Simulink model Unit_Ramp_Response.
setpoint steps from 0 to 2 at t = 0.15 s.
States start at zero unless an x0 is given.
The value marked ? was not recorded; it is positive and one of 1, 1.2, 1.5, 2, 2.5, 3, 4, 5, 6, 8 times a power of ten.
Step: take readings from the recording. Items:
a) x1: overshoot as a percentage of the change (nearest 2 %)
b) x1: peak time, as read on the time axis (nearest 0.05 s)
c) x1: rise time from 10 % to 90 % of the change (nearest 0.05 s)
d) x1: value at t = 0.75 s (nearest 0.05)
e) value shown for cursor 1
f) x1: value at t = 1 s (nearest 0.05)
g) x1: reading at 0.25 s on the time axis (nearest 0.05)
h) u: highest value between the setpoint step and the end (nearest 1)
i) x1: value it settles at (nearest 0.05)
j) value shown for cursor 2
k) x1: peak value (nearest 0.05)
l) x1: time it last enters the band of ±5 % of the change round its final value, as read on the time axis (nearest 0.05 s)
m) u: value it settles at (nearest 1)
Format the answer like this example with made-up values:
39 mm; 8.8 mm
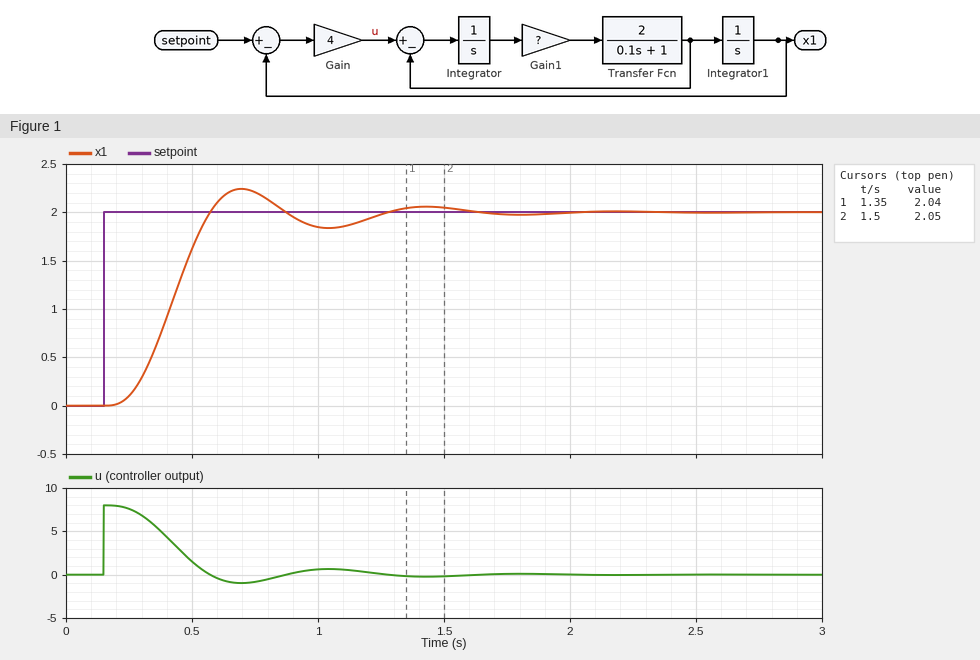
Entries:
12 %; 0.70 s; 0.25 s; 2.20; 2.04; 1.85; 0.10; 8; 2.00; 2.05; 2.25; 1.15 s; 0
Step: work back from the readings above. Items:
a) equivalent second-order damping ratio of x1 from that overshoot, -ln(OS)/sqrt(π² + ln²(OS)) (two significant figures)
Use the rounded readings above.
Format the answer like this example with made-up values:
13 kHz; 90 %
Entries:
0.56
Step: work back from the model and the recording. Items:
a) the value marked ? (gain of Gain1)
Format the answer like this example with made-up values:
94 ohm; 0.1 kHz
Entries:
5
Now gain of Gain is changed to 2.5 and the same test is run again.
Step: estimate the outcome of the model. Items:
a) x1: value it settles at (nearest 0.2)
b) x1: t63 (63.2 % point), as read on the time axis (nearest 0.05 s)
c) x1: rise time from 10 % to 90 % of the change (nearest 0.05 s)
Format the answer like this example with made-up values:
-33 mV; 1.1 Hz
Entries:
2.0; 0.55 s; 0.50 s
